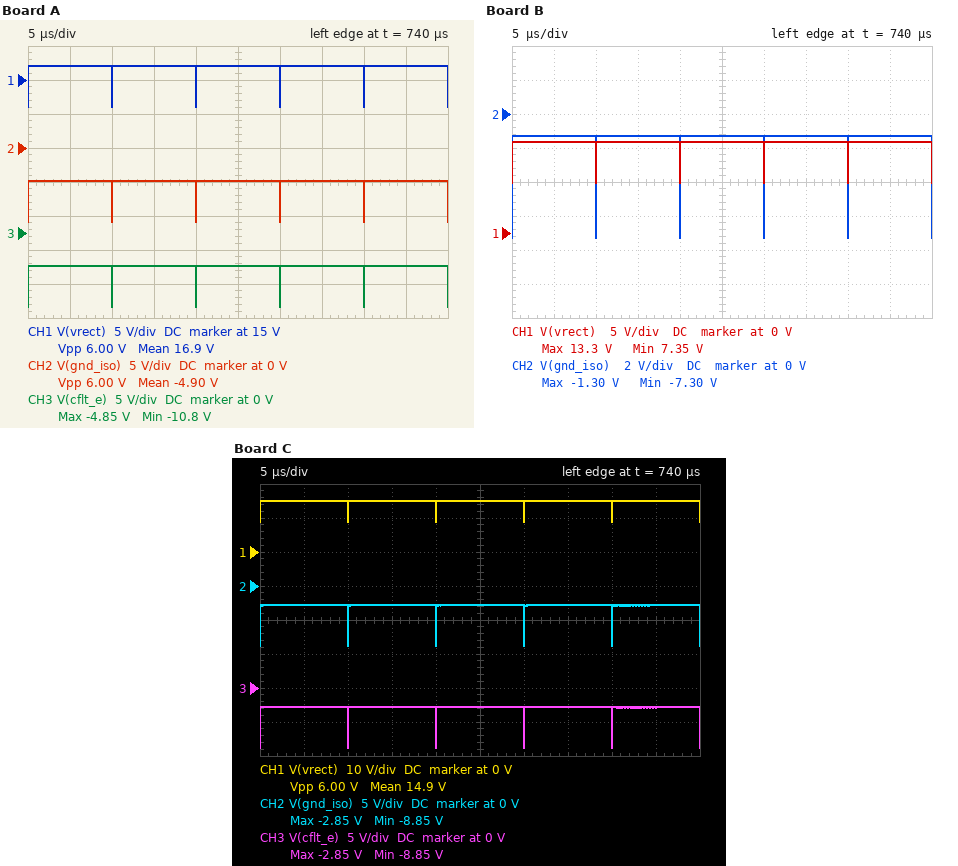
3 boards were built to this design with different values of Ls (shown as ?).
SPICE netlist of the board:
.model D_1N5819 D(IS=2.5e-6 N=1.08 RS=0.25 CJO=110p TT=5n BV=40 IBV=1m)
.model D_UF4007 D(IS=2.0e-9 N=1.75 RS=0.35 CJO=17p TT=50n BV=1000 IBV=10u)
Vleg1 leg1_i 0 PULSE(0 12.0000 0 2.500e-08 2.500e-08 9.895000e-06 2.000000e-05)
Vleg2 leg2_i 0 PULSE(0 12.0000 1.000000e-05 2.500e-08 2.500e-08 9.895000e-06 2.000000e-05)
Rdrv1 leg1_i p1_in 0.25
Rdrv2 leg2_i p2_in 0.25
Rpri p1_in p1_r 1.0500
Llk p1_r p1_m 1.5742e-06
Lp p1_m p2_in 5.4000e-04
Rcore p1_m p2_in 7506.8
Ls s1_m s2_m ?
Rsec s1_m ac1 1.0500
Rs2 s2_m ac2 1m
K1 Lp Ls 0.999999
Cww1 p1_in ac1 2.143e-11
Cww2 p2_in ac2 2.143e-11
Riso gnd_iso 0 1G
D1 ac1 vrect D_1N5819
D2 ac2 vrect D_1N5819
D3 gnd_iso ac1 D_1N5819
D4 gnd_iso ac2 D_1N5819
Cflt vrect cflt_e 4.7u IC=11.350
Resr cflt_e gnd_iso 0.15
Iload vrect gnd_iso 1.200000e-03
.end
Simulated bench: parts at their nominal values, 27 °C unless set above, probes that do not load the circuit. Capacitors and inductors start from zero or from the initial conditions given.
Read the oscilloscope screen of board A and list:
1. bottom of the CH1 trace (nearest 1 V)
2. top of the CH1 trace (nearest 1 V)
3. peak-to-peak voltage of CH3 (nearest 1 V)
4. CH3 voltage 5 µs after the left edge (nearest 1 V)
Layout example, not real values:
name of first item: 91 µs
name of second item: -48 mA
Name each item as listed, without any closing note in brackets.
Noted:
bottom of the CH1 trace: 11 V
top of the CH1 trace: 17 V
peak-to-peak voltage of CH3: 6 V
CH3 voltage 5 µs after the left edge: -5 V
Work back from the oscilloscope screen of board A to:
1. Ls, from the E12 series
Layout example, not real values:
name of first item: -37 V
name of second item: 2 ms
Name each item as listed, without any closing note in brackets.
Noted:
Ls, from the E12 series: 1.8 mH
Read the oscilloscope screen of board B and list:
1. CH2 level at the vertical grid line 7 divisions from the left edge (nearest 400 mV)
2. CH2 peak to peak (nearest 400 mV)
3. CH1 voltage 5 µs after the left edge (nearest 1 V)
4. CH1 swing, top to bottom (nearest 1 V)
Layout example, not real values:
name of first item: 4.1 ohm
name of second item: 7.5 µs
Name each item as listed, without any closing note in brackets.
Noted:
CH2 level at the vertical grid line 7 divisions from the left edge: -1.2 V
CH2 peak to peak: 6.0 V
CH1 voltage 5 µs after the left edge: 13 V
CH1 swing, top to bottom: 6 V
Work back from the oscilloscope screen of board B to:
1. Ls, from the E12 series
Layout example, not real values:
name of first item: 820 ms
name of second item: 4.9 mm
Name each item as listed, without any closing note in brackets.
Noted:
Ls, from the E12 series: 820 µH
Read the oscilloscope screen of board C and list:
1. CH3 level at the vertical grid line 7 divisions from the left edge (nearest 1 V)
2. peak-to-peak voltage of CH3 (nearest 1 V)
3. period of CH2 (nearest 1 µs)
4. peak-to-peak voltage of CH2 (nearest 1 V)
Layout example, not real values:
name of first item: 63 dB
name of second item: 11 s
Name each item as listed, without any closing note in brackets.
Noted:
CH3 level at the vertical grid line 7 divisions from the left edge: -3 V
peak-to-peak voltage of CH3: 6 V
period of CH2: 10 µs
peak-to-peak voltage of CH2: 6 V
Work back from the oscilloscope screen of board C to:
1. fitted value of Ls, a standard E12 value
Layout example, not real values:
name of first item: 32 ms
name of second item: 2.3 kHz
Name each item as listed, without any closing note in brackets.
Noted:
fitted value of Ls, a standard E12 value: 1.2 mH
